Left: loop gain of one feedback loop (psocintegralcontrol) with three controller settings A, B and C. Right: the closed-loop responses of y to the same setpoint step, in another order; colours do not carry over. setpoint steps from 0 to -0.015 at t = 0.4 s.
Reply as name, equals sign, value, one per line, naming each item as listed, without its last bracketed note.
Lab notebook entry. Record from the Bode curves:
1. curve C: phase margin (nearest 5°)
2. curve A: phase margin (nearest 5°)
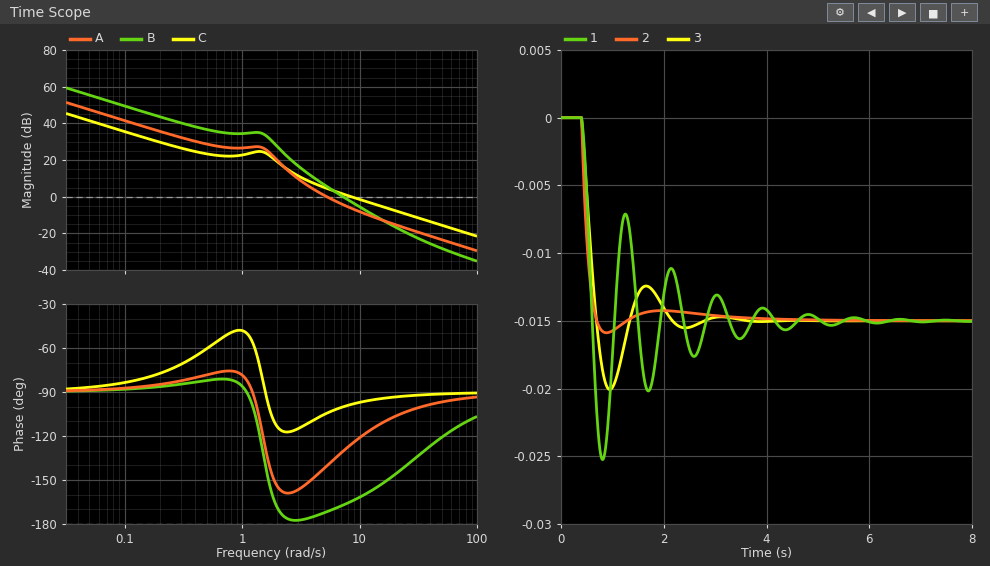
curve C: phase margin = 80°
curve A: phase margin = 40°
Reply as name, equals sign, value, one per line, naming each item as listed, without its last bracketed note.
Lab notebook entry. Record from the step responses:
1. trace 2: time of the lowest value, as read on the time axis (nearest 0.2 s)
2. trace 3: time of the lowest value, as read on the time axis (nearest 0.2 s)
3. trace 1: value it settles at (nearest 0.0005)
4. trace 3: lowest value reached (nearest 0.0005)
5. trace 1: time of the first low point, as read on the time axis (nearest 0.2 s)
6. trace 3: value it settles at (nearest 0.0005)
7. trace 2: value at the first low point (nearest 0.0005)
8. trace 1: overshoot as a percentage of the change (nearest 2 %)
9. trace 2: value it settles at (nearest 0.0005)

trace 2: time of the lowest value, as read on the time axis = 0.8 s
trace 3: time of the lowest value, as read on the time axis = 1.0 s
trace 1: value it settles at = -0.0150
trace 3: lowest value reached = -0.0200
trace 1: time of the first low point, as read on the time axis = 0.8 s
trace 3: value it settles at = -0.0150
trace 2: value at the first low point = -0.0160
trace 1: overshoot as a percentage of the change = 68 %
trace 2: value it settles at = -0.0150
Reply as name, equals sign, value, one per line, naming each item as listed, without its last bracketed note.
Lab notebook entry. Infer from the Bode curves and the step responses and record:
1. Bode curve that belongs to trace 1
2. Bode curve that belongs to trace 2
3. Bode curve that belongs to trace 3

Bode curve that belongs to trace 1 = B
Bode curve that belongs to trace 2 = C
Bode curve that belongs to trace 3 = A
